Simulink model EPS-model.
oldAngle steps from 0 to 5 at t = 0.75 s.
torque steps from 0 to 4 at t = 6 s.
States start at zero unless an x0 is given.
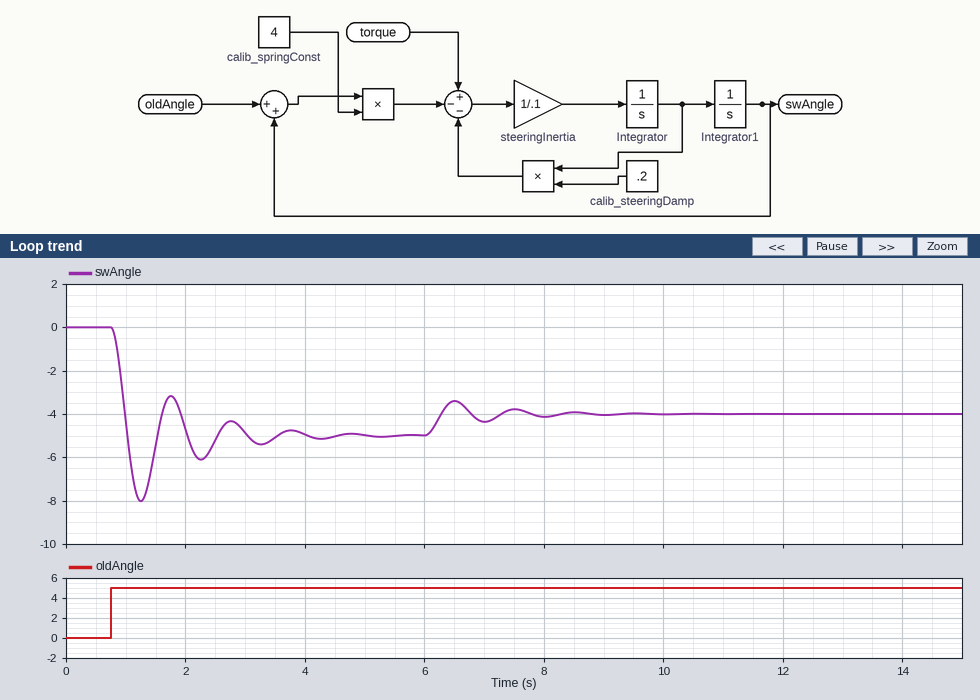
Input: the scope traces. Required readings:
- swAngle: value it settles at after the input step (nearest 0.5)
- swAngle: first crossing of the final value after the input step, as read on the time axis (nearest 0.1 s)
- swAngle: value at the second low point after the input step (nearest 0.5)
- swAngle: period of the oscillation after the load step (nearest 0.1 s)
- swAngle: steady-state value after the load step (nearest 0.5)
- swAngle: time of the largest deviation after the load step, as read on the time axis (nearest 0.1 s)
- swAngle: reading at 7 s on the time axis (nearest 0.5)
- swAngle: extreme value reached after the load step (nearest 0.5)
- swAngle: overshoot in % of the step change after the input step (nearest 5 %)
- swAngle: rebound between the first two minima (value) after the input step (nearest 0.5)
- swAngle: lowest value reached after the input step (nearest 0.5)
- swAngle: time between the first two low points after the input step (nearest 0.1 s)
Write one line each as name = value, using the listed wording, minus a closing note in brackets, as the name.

swAngle: value it settles at after the input step = -5.0
swAngle: first crossing of the final value after the input step, as read on the time axis = 1.0 s
swAngle: value at the second low point after the input step = -6.0
swAngle: period of the oscillation after the load step = 1.0 s
swAngle: steady-state value after the load step = -4.0
swAngle: time of the largest deviation after the load step, as read on the time axis = 6.5 s
swAngle: reading at 7 s on the time axis = -4.5
swAngle: extreme value reached after the load step = -3.5
swAngle: overshoot in % of the step change after the input step = 60 %
swAngle: rebound between the first two minima (value) after the input step = -3.0
swAngle: lowest value reached after the input step = -8.0
swAngle: time between the first two low points after the input step = 1.0 s
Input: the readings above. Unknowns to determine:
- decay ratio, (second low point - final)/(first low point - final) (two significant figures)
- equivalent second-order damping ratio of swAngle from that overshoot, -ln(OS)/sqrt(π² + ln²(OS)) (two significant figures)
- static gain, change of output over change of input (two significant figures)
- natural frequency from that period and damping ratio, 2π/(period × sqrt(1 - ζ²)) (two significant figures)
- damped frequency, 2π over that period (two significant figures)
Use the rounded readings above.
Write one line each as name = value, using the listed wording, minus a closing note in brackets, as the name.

decay ratio, (second low point - final)/(first low point - final) = 0.33
equivalent second-order damping ratio of swAngle from that overshoot, -ln(OS)/sqrt(π² + ln²(OS)) = 0.16
static gain, change of output over change of input = -1.0
natural frequency from that period and damping ratio, 2π/(period × sqrt(1 - ζ²)) = 6.4 rad/s
damped frequency, 2π over that period = 6.3 rad/s
